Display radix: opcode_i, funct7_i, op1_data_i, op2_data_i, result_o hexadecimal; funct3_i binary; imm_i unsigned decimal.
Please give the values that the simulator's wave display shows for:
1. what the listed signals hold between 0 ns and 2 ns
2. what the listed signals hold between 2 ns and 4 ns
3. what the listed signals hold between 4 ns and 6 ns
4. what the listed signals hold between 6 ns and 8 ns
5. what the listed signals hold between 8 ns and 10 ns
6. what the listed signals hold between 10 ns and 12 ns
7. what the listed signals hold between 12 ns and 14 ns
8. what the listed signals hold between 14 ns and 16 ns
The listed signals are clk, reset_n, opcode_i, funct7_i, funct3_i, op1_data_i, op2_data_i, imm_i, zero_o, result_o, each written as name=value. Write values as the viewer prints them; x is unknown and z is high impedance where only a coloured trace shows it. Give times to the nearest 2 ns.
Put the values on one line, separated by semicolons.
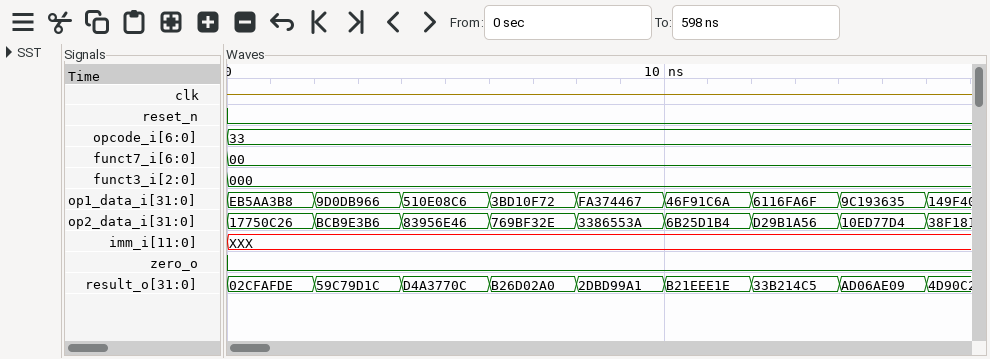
clk=z, reset_n=0, opcode_i=33, funct7_i=00, funct3_i=000, op1_data_i=EB5AA3B8, op2_data_i=17750C26, imm_i=XXX, zero_o=0, result_o=02CFAFDE; clk=z, reset_n=0, opcode_i=33, funct7_i=00, funct3_i=000, op1_data_i=9D0DB966, op2_data_i=BCB9E3B6, imm_i=XXX, zero_o=0, result_o=59C79D1C; clk=z, reset_n=0, opcode_i=33, funct7_i=00, funct3_i=000, op1_data_i=510E08C6, op2_data_i=83956E46, imm_i=XXX, zero_o=0, result_o=D4A3770C; clk=z, reset_n=0, opcode_i=33, funct7_i=00, funct3_i=000, op1_data_i=3BD10F72, op2_data_i=769BF32E, imm_i=XXX, zero_o=0, result_o=B26D02A0; clk=z, reset_n=0, opcode_i=33, funct7_i=00, funct3_i=000, op1_data_i=FA374467, op2_data_i=3386553A, imm_i=XXX, zero_o=0, result_o=2DBD99A1; clk=z, reset_n=0, opcode_i=33, funct7_i=00, funct3_i=000, op1_data_i=46F91C6A, op2_data_i=6B25D1B4, imm_i=XXX, zero_o=0, result_o=B21EEE1E; clk=z, reset_n=0, opcode_i=33, funct7_i=00, funct3_i=000, op1_data_i=6116FA6F, op2_data_i=D29B1A56, imm_i=XXX, zero_o=0, result_o=33B214C5; clk=z, reset_n=0, opcode_i=33, funct7_i=00, funct3_i=000, op1_data_i=9C193635, op2_data_i=10ED77D4, imm_i=XXX, zero_o=0, result_o=AD06AE09
